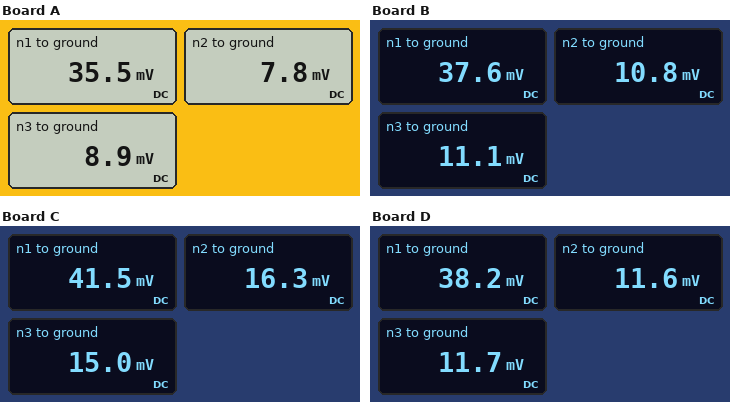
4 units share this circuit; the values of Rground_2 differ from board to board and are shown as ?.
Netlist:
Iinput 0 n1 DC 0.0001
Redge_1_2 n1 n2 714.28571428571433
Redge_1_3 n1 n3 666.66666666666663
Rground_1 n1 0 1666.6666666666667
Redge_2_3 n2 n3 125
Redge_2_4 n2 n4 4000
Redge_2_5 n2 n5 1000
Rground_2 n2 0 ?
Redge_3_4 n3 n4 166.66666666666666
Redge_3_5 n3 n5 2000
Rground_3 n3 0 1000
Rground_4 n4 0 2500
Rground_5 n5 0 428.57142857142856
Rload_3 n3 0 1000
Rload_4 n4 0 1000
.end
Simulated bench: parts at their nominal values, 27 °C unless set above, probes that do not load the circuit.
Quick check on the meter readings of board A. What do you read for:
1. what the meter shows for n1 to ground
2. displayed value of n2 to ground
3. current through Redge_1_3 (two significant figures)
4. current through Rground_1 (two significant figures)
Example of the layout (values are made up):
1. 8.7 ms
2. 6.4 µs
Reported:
1. 35.5 mV
2. 7.8 mV
3. 40 µA
4. 21 µA
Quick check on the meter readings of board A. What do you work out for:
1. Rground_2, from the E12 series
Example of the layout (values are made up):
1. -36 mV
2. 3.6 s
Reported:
1. 180 Ω
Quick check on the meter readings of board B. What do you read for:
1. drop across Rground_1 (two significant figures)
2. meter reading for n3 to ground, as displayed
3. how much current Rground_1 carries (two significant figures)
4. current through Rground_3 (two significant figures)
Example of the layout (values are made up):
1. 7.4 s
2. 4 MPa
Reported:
1. 38 mV
2. 11.1 mV
3. 23 µA
4. 11 µA
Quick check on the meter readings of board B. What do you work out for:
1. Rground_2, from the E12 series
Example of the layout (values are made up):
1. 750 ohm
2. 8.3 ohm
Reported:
1. 330 Ω
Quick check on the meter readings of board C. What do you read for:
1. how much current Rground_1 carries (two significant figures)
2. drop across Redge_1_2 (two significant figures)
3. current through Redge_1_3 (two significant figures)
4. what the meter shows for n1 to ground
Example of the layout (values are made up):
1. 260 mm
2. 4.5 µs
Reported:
1. 25 µA
2. 25 mV
3. 40 µA
4. 41.5 mV
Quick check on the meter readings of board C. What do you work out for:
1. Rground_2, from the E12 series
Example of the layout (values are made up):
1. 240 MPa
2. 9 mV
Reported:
1. 1.2 kΩ
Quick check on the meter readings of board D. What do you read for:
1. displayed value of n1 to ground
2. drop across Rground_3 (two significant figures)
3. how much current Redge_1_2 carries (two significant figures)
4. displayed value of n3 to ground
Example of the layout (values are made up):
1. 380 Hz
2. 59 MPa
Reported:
1. 38.2 mV
2. 12 mV
3. 37 µA
4. 11.7 mV
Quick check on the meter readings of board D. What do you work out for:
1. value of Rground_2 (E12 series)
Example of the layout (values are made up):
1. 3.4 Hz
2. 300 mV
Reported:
1. 390 Ω
